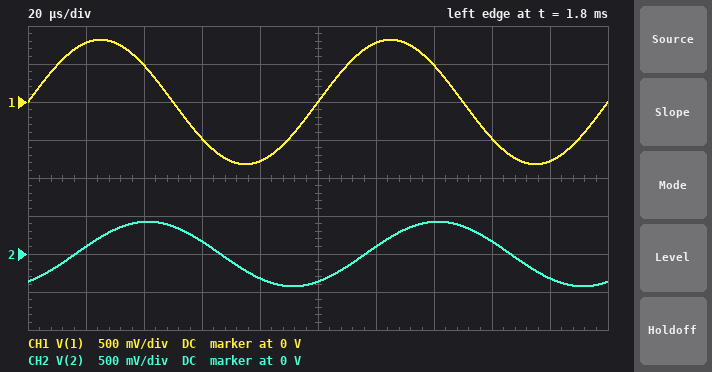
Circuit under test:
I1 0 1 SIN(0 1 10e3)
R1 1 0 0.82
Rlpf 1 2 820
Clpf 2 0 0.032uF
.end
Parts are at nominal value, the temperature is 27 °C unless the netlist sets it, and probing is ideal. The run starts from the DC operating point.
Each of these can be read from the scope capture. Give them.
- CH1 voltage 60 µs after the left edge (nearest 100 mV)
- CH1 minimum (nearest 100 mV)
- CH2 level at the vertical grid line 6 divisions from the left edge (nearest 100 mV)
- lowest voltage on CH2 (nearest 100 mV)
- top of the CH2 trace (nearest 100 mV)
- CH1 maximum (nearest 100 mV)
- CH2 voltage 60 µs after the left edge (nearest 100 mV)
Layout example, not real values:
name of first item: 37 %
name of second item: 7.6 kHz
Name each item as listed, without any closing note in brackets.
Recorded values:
CH1 voltage 60 µs after the left edge: -500 mV
CH1 minimum: -800 mV
CH2 level at the vertical grid line 6 divisions from the left edge: 100 mV
lowest voltage on CH2: -400 mV
top of the CH2 trace: 400 mV
CH1 maximum: 800 mV
CH2 voltage 60 µs after the left edge: 200 mV
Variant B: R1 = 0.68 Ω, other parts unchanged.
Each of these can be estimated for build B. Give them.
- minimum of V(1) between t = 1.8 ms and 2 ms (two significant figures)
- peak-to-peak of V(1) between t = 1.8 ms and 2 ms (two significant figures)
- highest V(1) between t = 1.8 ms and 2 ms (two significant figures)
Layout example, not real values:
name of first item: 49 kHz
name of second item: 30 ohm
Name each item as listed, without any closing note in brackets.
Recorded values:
minimum of V(1) between t = 1.8 ms and 2 ms: -680 mV
peak-to-peak of V(1) between t = 1.8 ms and 2 ms: 1.4 V
highest V(1) between t = 1.8 ms and 2 ms: 680 mV
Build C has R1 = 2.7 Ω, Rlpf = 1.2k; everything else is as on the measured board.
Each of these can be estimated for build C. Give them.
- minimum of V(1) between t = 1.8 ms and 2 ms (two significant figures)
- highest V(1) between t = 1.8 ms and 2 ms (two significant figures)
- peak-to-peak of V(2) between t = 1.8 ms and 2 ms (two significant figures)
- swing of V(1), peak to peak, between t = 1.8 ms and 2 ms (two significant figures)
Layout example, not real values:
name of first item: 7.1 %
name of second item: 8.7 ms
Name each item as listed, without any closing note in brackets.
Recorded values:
minimum of V(1) between t = 1.8 ms and 2 ms: -2.7 V
highest V(1) between t = 1.8 ms and 2 ms: 2.7 V
peak-to-peak of V(2) between t = 1.8 ms and 2 ms: 2.1 V
swing of V(1), peak to peak, between t = 1.8 ms and 2 ms: 5.4 V
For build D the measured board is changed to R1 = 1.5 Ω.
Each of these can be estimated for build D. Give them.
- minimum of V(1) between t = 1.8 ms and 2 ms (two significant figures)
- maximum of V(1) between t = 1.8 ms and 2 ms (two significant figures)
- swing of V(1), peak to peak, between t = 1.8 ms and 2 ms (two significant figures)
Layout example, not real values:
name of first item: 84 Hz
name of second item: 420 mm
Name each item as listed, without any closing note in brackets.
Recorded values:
minimum of V(1) between t = 1.8 ms and 2 ms: -1.5 V
maximum of V(1) between t = 1.8 ms and 2 ms: 1.5 V
swing of V(1), peak to peak, between t = 1.8 ms and 2 ms: 3.0 V
